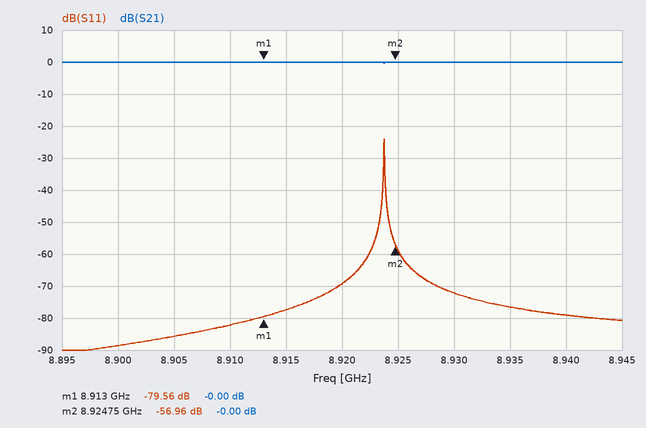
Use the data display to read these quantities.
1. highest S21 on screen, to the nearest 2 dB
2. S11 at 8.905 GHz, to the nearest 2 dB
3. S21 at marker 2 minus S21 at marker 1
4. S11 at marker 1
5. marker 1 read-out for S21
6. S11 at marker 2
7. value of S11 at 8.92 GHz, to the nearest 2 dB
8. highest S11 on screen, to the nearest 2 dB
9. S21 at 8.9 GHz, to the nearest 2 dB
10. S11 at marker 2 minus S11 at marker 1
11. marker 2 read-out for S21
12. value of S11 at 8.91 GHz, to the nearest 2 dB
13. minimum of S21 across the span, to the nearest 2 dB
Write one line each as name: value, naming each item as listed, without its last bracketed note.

highest S21 on screen, to the nearest 2 dB: 0 dB
S11 at 8.905 GHz, to the nearest 2 dB: -86 dB
S21 at marker 2 minus S21 at marker 1: 0.00 dB
S11 at marker 1: -79.56 dB
marker 1 read-out for S21: -0.00 dB
S11 at marker 2: -56.96 dB
value of S11 at 8.92 GHz, to the nearest 2 dB: -70 dB
highest S11 on screen, to the nearest 2 dB: -24 dB
S21 at 8.9 GHz, to the nearest 2 dB: 0 dB
S11 at marker 2 minus S11 at marker 1: 22.60 dB
marker 2 read-out for S21: -0.00 dB
value of S11 at 8.91 GHz, to the nearest 2 dB: -82 dB
minimum of S21 across the span, to the nearest 2 dB: 0 dB
